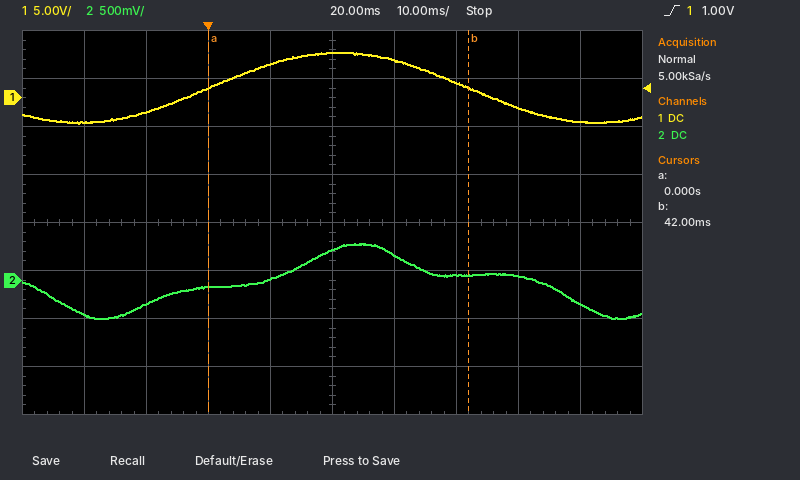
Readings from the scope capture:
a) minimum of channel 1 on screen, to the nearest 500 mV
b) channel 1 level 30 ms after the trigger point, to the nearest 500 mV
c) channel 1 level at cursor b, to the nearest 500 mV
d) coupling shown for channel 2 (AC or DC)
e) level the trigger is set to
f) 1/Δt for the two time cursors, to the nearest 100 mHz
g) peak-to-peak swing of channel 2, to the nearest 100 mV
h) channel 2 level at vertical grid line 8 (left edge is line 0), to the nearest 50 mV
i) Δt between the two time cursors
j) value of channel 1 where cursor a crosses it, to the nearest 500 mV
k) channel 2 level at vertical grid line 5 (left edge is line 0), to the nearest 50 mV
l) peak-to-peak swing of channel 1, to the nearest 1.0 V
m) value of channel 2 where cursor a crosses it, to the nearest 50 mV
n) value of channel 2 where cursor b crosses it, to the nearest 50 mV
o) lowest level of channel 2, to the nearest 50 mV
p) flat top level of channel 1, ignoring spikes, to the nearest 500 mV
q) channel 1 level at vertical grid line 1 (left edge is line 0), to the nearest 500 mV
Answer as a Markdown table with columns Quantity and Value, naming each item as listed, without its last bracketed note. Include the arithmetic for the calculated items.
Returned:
| Quantity | Value |
|---|---|
| minimum of channel 1 on screen, to the nearest 500 mV | -2.5 V |
| channel 1 level 30 ms after the trigger point, to the nearest 500 mV | 4.0 V |
| channel 1 level at cursor b, to the nearest 500 mV | 1.0 V |
| coupling shown for channel 2 | DC |
| level the trigger is set to | 1.00 V |
| 1/Δt for the two time cursors, to the nearest 100 mHz | 1 / 42 ms ≈ 23.8 Hz |
| peak-to-peak swing of channel 2, to the nearest 100 mV | 800 mV |
| channel 2 level at vertical grid line 8 (left edge is line 0), to the nearest 50 mV | 50 mV |
| Δt between the two time cursors | 42 ms − (0 s) = 42 ms |
| value of channel 1 where cursor a crosses it, to the nearest 500 mV | 1.0 V |
| channel 2 level at vertical grid line 5 (left edge is line 0), to the nearest 50 mV | 300 mV |
| peak-to-peak swing of channel 1, to the nearest 1.0 V | 7.0 V |
| value of channel 2 where cursor a crosses it, to the nearest 50 mV | -50 mV |
| value of channel 2 where cursor b crosses it, to the nearest 50 mV | 50 mV |
| lowest level of channel 2, to the nearest 50 mV | -400 mV |
| flat top level of channel 1, ignoring spikes, to the nearest 500 mV | 4.5 V |
| channel 1 level at vertical grid line 1 (left edge is line 0), to the nearest 500 mV | -2.5 V |
